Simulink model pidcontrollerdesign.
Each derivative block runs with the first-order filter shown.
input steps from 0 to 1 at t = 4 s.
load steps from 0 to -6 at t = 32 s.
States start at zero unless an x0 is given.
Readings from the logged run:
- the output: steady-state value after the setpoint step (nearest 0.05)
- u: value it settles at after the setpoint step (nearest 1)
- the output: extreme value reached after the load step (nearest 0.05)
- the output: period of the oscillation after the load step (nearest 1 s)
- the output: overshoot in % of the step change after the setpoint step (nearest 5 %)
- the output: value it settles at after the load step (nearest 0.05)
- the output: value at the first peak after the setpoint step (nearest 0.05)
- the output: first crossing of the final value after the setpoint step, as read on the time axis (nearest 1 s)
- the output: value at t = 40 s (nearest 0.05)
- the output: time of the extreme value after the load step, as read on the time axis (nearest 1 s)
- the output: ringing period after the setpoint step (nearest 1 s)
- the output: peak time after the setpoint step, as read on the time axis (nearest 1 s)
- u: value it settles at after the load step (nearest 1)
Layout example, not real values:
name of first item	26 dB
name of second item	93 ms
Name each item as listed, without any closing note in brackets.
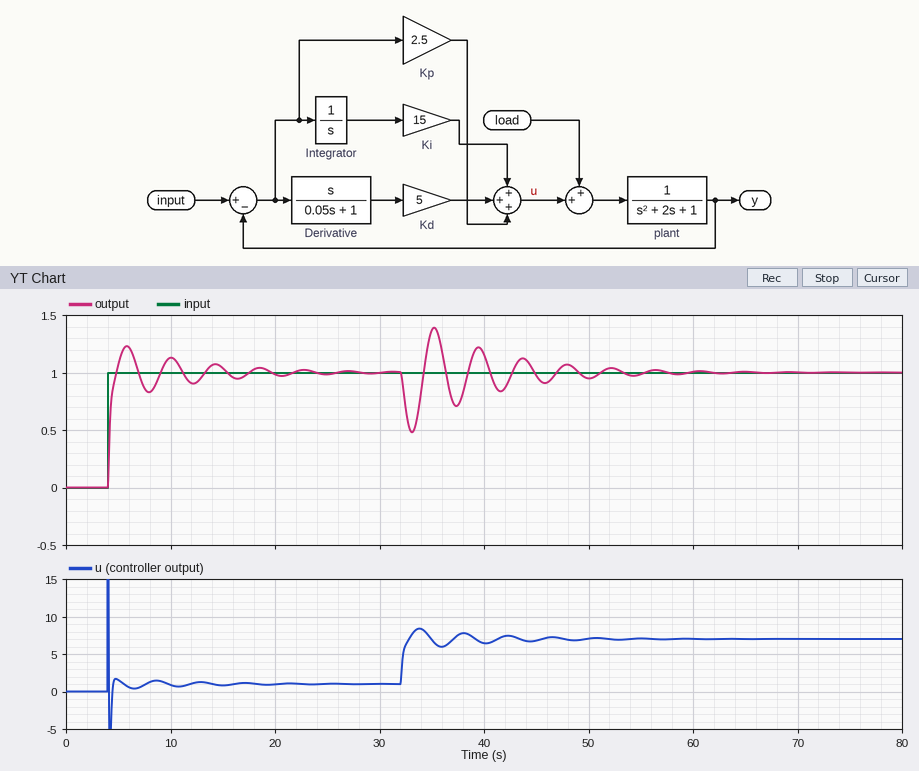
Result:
the output: steady-state value after the setpoint step	1.00
u: value it settles at after the setpoint step	1
the output: extreme value reached after the load step	0.50
the output: period of the oscillation after the load step	4 s
the output: overshoot in % of the step change after the setpoint step	25 %
the output: value it settles at after the load step	1.00
the output: value at the first peak after the setpoint step	1.25
the output: first crossing of the final value after the setpoint step, as read on the time axis	5 s
the output: value at t = 40 s	1.15
the output: time of the extreme value after the load step, as read on the time axis	33 s
the output: ringing period after the setpoint step	4 s
the output: peak time after the setpoint step, as read on the time axis	6 s
u: value it settles at after the load step	7
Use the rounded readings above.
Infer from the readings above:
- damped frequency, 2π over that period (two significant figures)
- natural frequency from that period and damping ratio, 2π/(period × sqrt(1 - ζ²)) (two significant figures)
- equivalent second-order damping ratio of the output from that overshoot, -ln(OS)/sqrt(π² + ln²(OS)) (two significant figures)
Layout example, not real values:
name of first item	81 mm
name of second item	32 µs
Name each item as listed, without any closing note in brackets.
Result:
damped frequency, 2π over that period	1.6 rad/s
natural frequency from that period and damping ratio, 2π/(period × sqrt(1 - ζ²))	1.7 rad/s
equivalent second-order damping ratio of the output from that overshoot, -ln(OS)/sqrt(π² + ln²(OS))	0.40
